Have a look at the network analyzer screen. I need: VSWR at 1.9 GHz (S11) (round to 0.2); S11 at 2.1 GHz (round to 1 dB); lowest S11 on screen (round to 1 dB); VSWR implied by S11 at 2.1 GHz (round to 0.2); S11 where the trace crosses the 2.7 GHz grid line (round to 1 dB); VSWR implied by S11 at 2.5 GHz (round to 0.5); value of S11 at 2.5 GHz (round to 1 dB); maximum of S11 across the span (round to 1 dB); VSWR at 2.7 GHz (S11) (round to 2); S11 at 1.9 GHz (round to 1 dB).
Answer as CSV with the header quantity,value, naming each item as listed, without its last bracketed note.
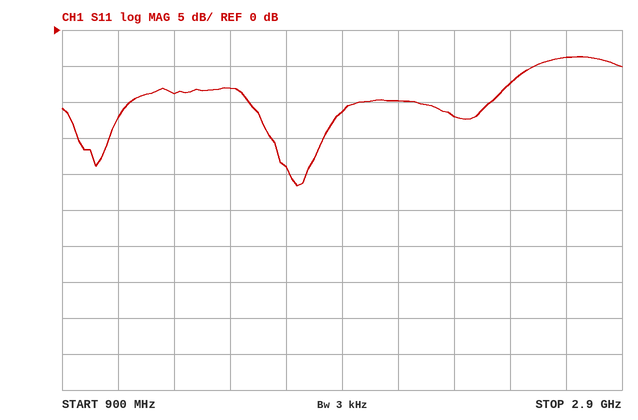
quantity,value
VSWR at 1.9 GHz (S11),1.8
S11 at 2.1 GHz,-10 dB
lowest S11 on screen,-22 dB
VSWR implied by S11 at 2.1 GHz,2.0
S11 where the trace crosses the 2.7 GHz grid line,-4 dB
VSWR implied by S11 at 2.5 GHz,2.5
value of S11 at 2.5 GHz,-7 dB
maximum of S11 across the span,-4 dB
VSWR at 2.7 GHz (S11),4
S11 at 1.9 GHz,-11 dB
